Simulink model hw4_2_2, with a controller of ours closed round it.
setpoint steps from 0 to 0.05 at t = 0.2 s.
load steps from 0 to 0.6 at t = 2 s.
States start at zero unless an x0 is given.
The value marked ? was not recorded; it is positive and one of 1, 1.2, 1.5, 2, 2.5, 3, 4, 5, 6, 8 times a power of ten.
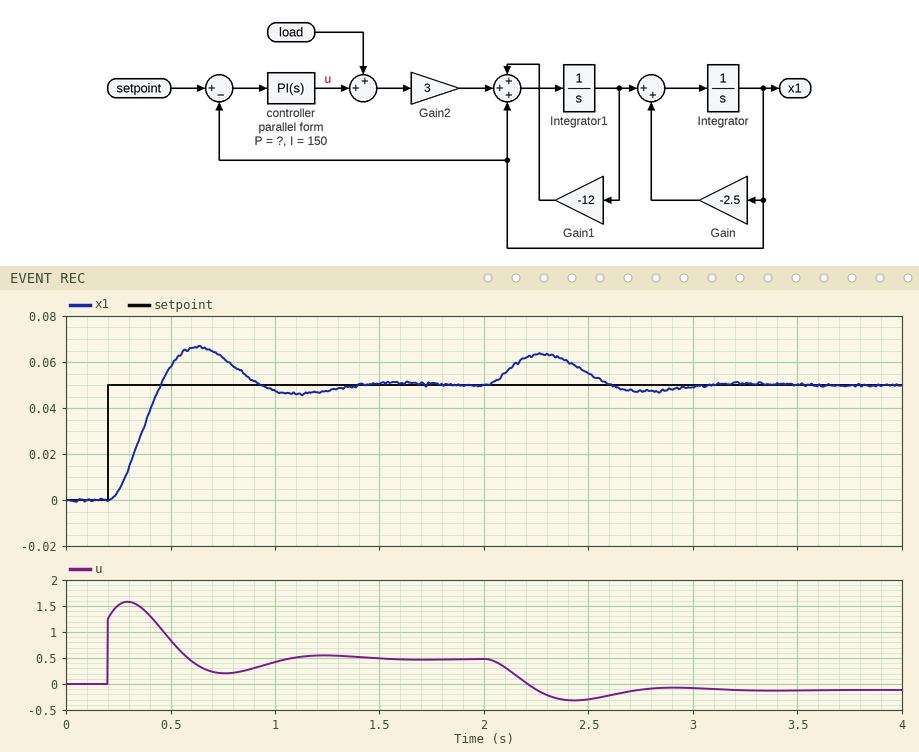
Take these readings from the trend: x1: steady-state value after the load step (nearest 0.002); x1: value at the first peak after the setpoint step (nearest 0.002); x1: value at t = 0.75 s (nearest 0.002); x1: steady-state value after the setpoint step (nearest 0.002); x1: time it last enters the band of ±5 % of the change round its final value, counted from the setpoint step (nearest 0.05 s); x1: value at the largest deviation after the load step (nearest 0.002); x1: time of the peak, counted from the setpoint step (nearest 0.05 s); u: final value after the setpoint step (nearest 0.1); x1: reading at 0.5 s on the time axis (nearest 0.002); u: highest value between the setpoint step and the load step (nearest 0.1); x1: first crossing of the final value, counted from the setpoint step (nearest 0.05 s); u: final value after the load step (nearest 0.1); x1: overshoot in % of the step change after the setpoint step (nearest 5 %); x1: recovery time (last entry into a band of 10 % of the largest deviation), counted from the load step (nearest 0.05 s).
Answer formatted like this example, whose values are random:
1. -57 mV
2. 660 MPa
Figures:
1. 0.050
2. 0.066
3. 0.062
4. 0.050
5. 1.05 s
6. 0.064
7. 0.45 s
8. 0.5
9. 0.058
10. 1.6
11. 0.25 s
12. -0.1
13. 35 %
14. 0.95 s
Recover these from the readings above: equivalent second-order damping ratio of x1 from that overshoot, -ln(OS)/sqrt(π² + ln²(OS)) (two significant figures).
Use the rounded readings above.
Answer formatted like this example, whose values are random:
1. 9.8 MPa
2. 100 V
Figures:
1. 0.32
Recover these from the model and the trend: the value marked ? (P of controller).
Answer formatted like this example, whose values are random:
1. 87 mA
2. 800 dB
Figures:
1. 25
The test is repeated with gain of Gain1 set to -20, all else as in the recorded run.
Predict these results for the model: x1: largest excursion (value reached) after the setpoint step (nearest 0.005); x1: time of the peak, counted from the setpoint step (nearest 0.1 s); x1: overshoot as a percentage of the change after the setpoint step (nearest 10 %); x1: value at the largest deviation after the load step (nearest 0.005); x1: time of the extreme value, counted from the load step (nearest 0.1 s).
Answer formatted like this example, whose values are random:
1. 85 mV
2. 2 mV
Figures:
1. 0.060
2. 0.6 s
3. 20 %
4. 0.060
5. 0.3 s
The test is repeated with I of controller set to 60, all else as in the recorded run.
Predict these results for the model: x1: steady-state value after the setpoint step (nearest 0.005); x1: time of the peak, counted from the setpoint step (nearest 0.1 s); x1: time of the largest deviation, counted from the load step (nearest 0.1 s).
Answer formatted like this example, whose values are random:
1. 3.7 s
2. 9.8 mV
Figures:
1. 0.050
2. 0.5 s
3. 0.3 s
